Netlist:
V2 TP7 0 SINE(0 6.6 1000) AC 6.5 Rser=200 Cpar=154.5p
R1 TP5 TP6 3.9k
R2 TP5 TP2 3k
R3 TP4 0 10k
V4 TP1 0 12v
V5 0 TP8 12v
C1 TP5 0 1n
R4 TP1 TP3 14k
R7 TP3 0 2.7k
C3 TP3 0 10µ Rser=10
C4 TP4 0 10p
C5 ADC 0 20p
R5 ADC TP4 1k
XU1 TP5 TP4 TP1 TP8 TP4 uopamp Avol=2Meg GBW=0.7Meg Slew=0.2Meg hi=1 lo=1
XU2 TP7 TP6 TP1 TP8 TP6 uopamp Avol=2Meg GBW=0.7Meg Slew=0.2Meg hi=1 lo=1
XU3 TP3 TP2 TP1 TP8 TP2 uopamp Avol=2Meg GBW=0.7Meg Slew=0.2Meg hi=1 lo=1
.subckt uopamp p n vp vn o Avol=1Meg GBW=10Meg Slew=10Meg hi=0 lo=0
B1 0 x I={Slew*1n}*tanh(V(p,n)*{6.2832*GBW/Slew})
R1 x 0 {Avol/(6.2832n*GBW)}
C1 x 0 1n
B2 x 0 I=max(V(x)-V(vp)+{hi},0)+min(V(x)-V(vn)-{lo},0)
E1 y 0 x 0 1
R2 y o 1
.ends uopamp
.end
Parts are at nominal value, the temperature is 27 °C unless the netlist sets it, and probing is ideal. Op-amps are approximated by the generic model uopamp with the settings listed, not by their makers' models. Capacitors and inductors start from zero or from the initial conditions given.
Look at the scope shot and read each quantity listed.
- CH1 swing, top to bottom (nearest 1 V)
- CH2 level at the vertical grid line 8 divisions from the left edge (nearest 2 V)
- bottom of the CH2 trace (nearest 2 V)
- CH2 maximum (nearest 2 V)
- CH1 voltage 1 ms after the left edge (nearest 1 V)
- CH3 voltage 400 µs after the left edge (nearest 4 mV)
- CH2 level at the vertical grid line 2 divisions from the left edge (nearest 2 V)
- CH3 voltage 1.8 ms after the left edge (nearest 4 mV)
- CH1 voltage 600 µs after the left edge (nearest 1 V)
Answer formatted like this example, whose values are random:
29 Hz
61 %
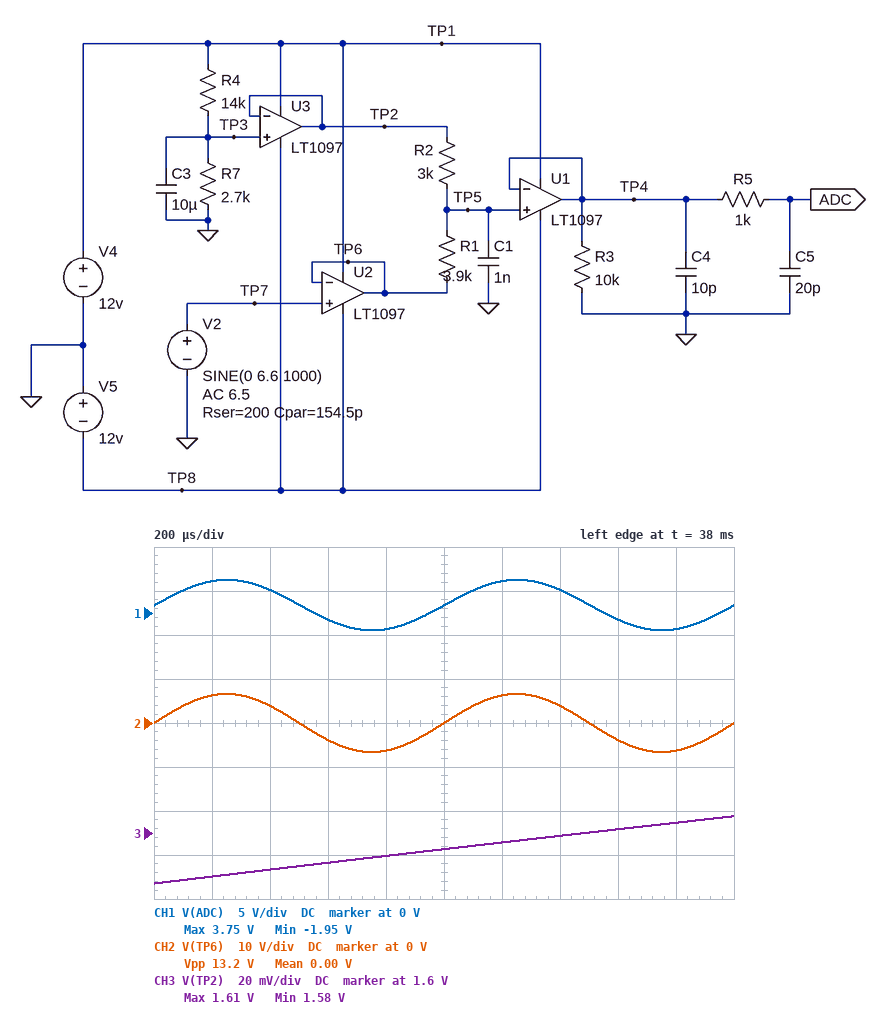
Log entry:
6 V
-4 V
-6 V
6 V
1 V
1.584 V
4 V
1.604 V
-1 V
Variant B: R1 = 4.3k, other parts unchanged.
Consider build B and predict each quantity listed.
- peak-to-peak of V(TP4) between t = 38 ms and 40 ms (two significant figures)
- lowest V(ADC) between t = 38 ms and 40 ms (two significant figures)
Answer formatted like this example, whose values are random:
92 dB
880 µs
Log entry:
5.4 V
-1.8 V
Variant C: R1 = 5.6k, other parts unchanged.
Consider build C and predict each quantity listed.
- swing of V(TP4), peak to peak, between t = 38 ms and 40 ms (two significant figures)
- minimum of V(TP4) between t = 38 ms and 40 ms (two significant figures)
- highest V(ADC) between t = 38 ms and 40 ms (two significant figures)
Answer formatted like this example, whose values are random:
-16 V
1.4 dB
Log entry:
4.6 V
-1.3 V
3.3 V
